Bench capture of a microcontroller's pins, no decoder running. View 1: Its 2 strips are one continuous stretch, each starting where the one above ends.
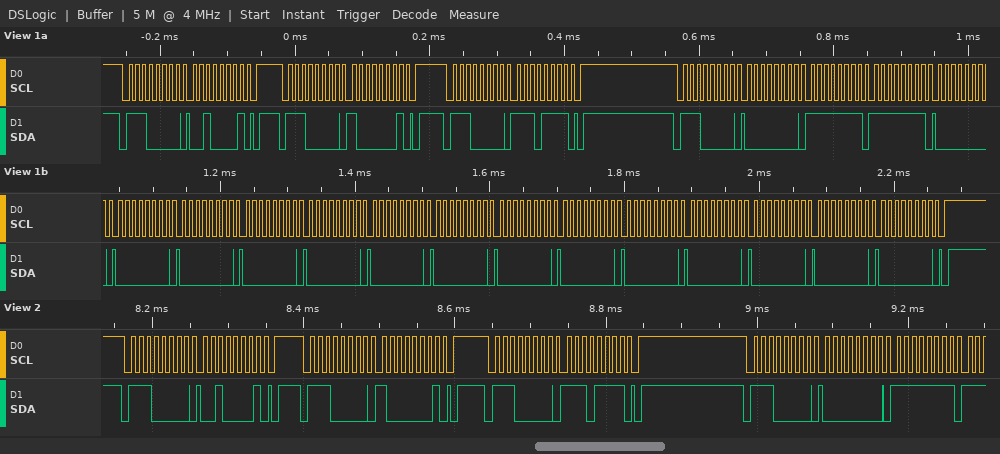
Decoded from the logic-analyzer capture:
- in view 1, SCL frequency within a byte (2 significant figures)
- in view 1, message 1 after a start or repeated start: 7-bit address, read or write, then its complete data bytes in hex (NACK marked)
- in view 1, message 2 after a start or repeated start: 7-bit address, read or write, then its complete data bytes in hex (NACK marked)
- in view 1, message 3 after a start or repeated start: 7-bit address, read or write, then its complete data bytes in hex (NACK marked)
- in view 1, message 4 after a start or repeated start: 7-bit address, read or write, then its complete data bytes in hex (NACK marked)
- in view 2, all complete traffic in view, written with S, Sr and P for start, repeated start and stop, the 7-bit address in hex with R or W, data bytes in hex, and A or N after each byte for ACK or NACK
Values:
100 kHz
0x70 write: 21
0x70 write: 81
0x70 write: EF
0x70 write: 00 FF FF 00 00 00 00 00 00 00 00 00 00 00 00 00 00
S 70W A 21 A P S 70W A 81 A P S 70W A EF A P S 70W A 00 A FF A
